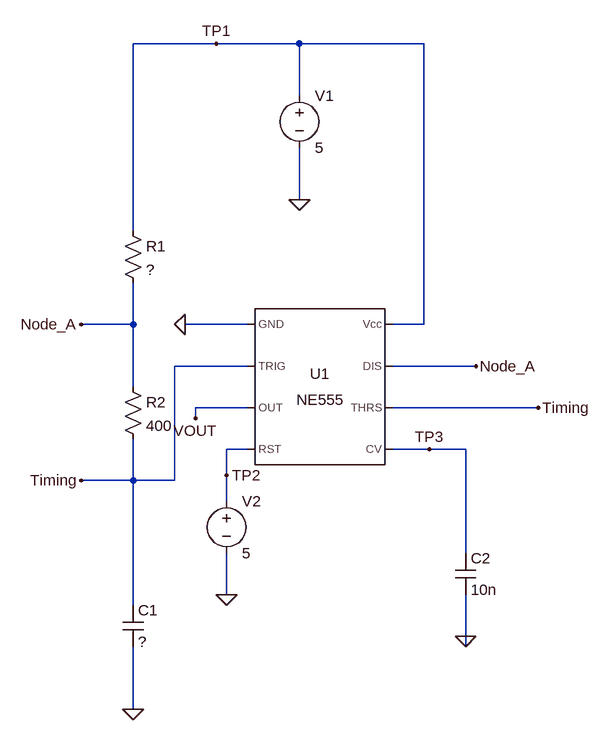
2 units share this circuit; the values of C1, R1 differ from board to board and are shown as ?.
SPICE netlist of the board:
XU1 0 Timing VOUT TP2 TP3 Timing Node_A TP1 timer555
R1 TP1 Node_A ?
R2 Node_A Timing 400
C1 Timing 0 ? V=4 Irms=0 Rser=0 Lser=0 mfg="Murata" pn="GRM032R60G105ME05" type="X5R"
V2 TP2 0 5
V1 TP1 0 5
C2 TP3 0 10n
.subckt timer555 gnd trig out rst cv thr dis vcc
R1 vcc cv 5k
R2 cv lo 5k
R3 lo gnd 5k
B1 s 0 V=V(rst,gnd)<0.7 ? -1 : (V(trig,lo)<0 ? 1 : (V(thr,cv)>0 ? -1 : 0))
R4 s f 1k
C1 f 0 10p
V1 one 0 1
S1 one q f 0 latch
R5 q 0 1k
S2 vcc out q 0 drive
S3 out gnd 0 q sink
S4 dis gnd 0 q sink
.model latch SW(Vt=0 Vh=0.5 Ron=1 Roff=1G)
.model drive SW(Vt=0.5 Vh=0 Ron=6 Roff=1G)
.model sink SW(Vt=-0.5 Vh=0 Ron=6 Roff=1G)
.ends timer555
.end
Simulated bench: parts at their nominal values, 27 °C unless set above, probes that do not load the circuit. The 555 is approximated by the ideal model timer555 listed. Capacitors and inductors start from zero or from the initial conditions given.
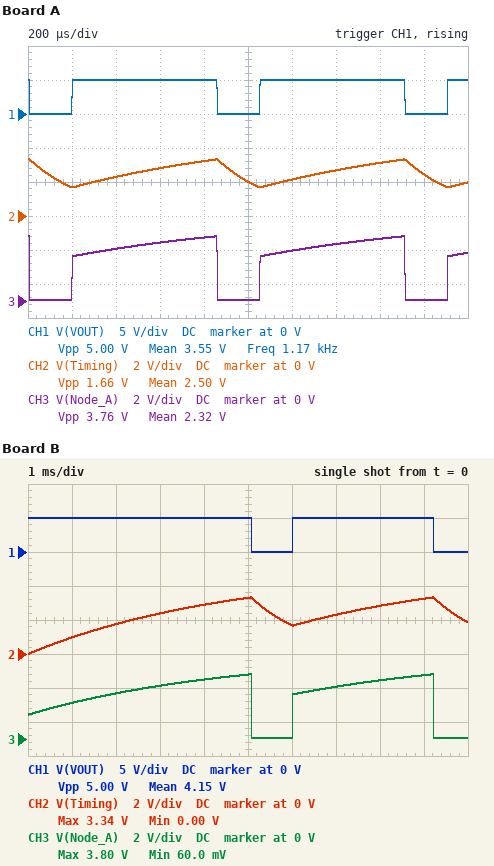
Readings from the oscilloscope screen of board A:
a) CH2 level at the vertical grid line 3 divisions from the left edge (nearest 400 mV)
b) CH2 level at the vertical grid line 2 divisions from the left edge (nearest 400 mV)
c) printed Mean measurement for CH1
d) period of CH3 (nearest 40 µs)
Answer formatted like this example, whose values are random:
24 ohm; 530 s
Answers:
2.8 V; 2.4 V; 3.55 V; 840 µs
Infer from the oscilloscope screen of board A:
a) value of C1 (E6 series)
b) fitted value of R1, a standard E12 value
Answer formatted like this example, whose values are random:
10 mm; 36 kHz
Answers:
680 nF; 1 kΩ
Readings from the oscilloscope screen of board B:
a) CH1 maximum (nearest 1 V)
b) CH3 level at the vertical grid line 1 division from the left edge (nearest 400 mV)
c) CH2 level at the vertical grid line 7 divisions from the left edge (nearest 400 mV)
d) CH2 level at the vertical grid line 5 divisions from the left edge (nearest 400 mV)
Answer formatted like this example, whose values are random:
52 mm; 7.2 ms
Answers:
5 V; 2.0 V; 2.4 V; 3.2 V
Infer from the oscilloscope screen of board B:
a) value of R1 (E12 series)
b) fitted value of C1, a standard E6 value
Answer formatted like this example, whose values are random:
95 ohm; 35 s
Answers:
1 kΩ; 3.3 µF
